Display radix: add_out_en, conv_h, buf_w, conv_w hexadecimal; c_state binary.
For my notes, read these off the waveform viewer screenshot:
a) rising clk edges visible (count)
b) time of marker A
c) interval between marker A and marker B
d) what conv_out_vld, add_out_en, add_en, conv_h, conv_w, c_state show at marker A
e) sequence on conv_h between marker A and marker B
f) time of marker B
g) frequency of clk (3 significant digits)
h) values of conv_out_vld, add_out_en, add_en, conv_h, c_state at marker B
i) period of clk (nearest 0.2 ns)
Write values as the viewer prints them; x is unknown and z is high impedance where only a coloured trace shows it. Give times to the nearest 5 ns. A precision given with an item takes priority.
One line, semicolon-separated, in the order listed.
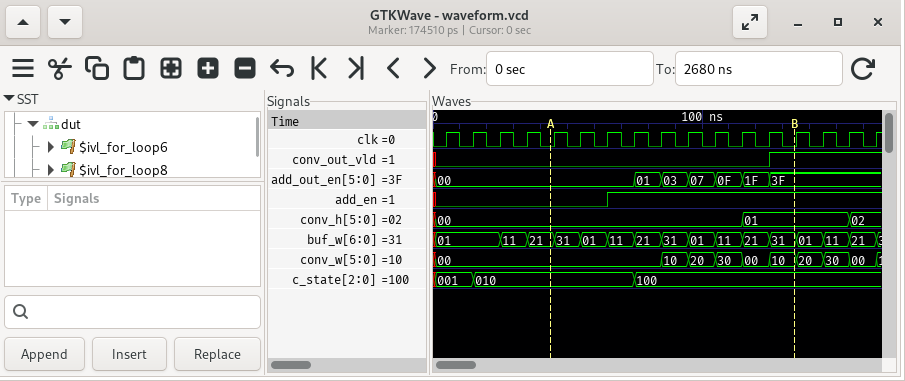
17; 45 ns; 90 ns; conv_out_vld=0, add_out_en=00, add_en=0, conv_h=00, conv_w=00, c_state=010; 00, 01; 135 ns; 100 MHz; conv_out_vld=1, add_out_en=3F, add_en=1, conv_h=01, c_state=100; 10 ns
